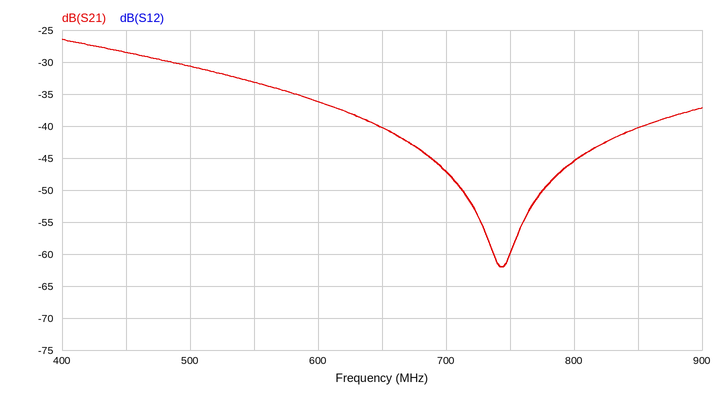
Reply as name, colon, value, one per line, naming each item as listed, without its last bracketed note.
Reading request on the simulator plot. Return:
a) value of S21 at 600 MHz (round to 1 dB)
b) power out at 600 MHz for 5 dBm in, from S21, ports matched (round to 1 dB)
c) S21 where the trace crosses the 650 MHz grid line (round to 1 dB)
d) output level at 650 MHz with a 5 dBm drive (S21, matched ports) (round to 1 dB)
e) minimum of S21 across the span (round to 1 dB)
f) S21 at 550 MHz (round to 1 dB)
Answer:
value of S21 at 600 MHz: -36 dB
power out at 600 MHz for 5 dBm in, from S21, ports matched: -31 dBm
S21 where the trace crosses the 650 MHz grid line: -40 dB
output level at 650 MHz with a 5 dBm drive (S21, matched ports): -35 dBm
minimum of S21 across the span: -62 dB
S21 at 550 MHz: -33 dB
